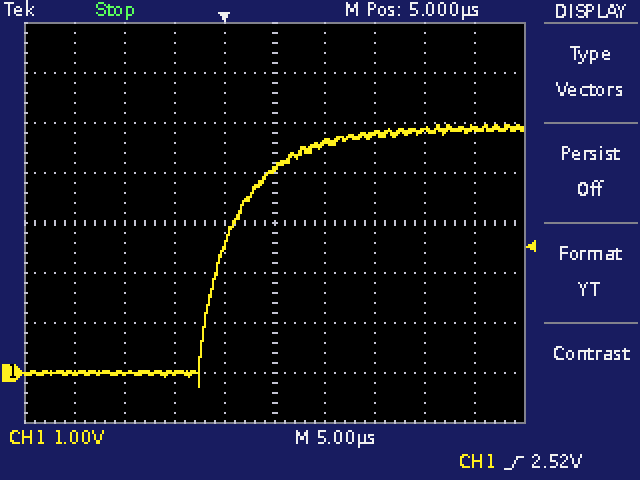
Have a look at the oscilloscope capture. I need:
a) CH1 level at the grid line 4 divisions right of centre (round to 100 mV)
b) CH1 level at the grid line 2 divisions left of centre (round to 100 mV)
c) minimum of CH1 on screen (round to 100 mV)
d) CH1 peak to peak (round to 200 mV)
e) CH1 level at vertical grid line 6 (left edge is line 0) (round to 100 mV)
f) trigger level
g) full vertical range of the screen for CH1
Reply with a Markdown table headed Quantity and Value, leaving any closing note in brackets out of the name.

| Quantity | Value |
|---|---|
| CH1 level at the grid line 4 divisions right of centre | 4.9 V |
| CH1 level at the grid line 2 divisions left of centre | 0.0 V |
| minimum of CH1 on screen | -300 mV |
| CH1 peak to peak | 5.2 V |
| CH1 level at vertical grid line 6 (left edge is line 0) | 4.6 V |
| trigger level | 2.52 V |
| full vertical range of the screen for CH1 | 8 V |
